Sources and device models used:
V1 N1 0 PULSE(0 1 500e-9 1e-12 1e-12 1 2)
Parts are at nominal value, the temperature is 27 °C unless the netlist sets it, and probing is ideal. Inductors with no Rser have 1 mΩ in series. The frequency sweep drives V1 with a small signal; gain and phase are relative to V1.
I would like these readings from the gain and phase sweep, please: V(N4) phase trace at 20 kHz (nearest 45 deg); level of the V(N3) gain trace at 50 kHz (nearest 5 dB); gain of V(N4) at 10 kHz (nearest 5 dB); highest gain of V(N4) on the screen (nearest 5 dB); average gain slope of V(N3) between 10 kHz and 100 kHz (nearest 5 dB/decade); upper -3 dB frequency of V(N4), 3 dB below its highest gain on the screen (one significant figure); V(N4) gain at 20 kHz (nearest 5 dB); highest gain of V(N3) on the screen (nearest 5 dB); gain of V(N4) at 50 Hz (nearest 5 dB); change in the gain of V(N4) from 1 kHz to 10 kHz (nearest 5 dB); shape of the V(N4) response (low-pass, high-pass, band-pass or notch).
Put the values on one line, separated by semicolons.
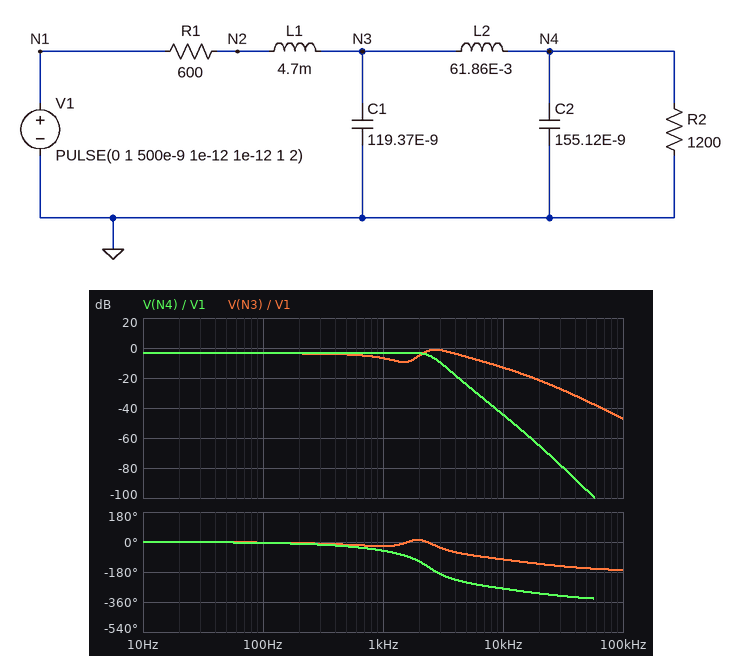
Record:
-315 deg; -35 dB; -45 dB; -5 dB; -35 dB/decade; 3 kHz; -65 dB; 0 dB; -5 dB; -40 dB; low-pass
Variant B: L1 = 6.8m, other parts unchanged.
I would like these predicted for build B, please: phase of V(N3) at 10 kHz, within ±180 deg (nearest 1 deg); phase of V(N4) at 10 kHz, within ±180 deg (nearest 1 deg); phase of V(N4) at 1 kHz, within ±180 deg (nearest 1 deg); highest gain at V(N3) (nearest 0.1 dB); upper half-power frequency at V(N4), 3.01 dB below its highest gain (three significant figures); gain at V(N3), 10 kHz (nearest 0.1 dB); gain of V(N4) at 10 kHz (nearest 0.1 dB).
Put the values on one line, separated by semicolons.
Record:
-116 deg; 69 deg; -53 deg; -1.0 dB; 2.64 kHz; -13.7 dB; -45.0 dB
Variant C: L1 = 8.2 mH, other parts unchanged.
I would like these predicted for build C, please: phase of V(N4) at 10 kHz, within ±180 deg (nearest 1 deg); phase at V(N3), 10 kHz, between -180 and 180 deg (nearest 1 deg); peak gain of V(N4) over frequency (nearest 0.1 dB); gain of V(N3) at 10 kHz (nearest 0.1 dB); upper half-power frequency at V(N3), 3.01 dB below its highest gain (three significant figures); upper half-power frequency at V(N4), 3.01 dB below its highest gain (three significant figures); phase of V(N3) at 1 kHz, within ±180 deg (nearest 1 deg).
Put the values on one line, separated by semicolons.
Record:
63 deg; -122 deg; -3.5 dB; -14.2 dB; 4.26 kHz; 2.65 kHz; -26 deg
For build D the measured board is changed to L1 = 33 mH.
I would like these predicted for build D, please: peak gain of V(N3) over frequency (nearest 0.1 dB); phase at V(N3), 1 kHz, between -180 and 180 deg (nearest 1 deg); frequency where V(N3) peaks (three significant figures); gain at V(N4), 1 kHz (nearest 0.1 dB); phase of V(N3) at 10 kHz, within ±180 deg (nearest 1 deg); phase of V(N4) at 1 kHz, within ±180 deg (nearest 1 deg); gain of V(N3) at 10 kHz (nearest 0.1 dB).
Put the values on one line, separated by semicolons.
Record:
1.6 dB; -35 deg; 2.98 kHz; -3.4 dB; -163 deg; -63 deg; -23.3 dB
